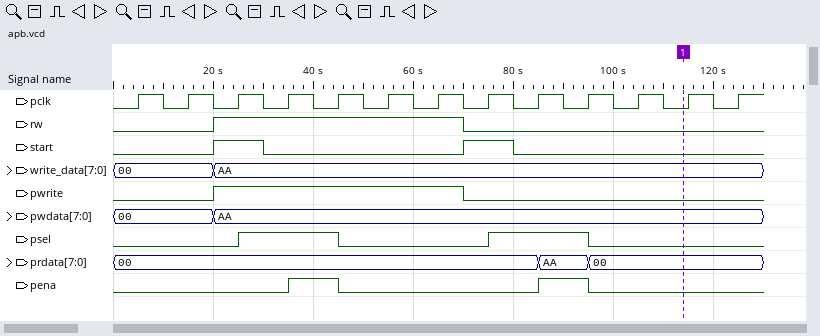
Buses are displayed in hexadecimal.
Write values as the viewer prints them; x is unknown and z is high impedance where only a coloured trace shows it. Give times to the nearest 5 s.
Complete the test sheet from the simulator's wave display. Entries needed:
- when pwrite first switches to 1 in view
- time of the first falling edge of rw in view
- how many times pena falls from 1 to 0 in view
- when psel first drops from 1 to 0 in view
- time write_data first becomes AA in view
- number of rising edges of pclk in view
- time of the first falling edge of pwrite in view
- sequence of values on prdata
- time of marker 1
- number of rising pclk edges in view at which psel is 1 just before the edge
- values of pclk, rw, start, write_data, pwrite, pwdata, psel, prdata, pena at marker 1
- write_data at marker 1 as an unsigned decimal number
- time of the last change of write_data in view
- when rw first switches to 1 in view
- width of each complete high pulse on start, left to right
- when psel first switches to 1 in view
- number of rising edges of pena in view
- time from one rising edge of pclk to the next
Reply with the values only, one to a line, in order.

20 s
70 s
2
45 s
20 s
13
70 s
00, AA, 00
115 s
4
pclk=0, rw=0, start=0, write_data=AA, pwrite=0, pwdata=AA, psel=0, prdata=00, pena=0
170
20 s
20 s
10 s, 10 s
25 s
2
10 s
